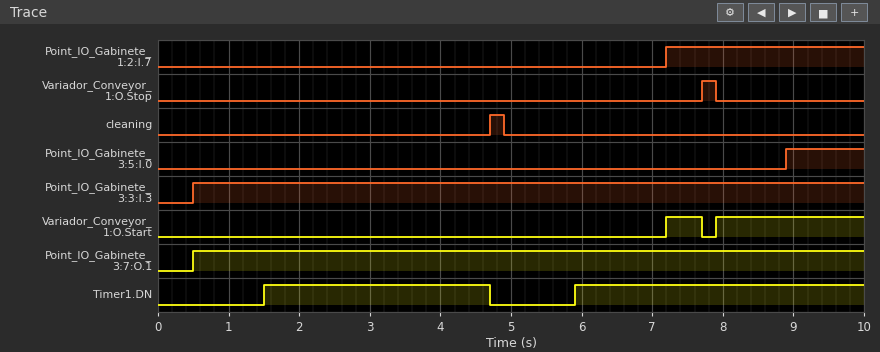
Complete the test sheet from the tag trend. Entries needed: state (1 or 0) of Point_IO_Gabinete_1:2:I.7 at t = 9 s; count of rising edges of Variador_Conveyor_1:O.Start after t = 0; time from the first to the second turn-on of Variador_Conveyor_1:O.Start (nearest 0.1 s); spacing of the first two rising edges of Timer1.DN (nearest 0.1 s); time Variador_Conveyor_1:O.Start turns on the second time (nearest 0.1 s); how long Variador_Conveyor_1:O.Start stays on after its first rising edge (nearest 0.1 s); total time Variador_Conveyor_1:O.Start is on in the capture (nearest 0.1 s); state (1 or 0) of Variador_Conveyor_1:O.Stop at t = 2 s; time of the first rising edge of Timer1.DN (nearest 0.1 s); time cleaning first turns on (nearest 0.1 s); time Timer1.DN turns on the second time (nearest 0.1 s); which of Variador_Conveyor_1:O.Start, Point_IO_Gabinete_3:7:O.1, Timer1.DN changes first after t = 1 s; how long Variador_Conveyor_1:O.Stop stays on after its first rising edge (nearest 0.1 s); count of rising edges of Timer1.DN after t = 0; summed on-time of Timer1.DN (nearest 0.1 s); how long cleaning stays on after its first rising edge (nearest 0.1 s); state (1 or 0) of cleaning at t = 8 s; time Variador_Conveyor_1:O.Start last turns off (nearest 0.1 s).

1
2
0.7 s
4.4 s
7.9 s
0.5 s
2.6 s
0
1.5 s
4.7 s
5.9 s
Timer1.DN
0.2 s
2
7.3 s
0.2 s
0
7.7 s
